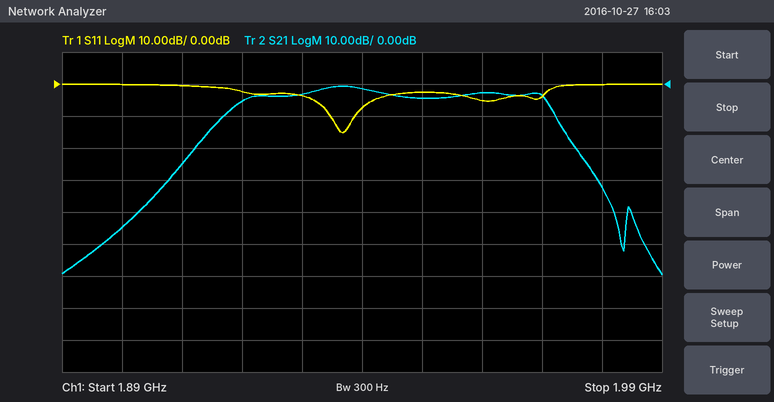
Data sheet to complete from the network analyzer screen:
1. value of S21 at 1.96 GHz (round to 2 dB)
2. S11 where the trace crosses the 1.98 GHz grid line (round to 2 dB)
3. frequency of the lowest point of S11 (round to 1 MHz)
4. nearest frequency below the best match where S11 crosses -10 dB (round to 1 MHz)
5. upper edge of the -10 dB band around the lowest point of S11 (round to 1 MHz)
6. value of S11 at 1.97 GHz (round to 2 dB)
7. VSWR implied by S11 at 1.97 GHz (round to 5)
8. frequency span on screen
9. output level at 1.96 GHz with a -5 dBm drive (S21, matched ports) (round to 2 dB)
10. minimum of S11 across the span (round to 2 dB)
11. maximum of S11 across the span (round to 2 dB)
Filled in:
-2 dB
0 dB
1.937 GHz
1.935 GHz
1.939 GHz
-4 dB
5
100 MHz
-8 dBm
-16 dB
0 dB
